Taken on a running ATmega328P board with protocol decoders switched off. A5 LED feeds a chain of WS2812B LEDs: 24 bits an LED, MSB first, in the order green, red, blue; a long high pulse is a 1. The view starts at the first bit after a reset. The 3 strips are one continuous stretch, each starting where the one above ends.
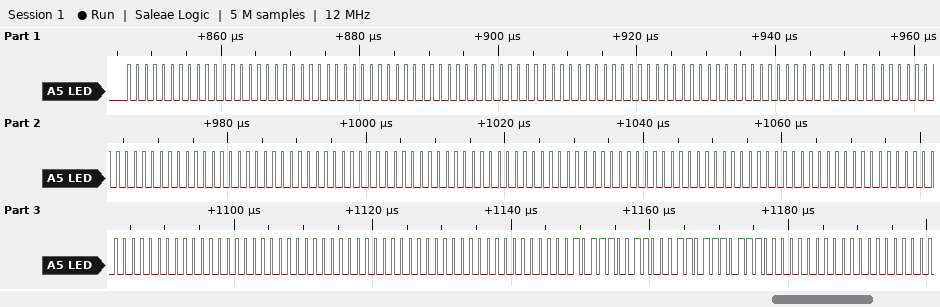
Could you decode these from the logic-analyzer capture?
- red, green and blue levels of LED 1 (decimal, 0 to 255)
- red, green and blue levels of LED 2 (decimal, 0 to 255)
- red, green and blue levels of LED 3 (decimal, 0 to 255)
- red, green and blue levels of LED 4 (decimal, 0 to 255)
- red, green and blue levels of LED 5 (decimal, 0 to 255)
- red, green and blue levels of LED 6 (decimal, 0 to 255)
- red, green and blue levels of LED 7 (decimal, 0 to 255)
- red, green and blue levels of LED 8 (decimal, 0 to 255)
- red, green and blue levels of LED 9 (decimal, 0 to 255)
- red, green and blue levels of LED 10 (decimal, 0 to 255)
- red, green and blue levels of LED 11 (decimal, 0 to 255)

0, 0, 0
0, 0, 0
0, 0, 0
0, 0, 0
0, 0, 0
0, 0, 0
0, 0, 0
0, 0, 0
0, 0, 0
0, 0, 0
99, 46, 119
